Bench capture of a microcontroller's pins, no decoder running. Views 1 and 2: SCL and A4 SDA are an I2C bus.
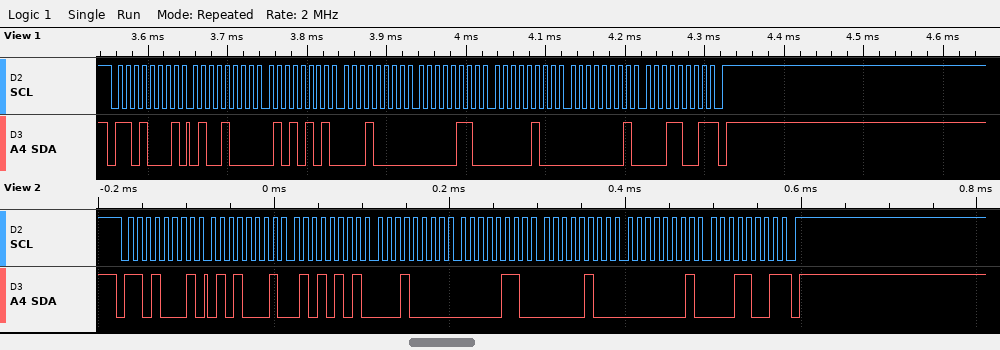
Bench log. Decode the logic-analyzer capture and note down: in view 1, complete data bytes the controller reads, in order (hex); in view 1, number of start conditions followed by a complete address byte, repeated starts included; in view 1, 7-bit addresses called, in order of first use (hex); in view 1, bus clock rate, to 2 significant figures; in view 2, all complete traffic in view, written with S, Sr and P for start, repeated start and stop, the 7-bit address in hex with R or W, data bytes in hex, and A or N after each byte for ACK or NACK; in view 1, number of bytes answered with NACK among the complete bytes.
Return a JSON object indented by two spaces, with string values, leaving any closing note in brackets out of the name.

{
  "in view 1, complete data bytes the controller reads, in order": "48 55 10 06 04 01 19",
  "in view 1, number of start conditions followed by a complete address byte, repeated starts included": "1",
  "in view 1, 7-bit addresses called, in order of first use": "0x68",
  "in view 1, bus clock rate, to 2 significant figures": "100 kHz",
  "in view 2, all complete traffic in view, written with S, Sr and P for start, repeated start and stop, the 7-bit address in hex with R or W, data bytes in hex, and A or N after each byte for ACK or NACK": "S 68R A 51 A 55 A 10 A 06 A 04 A 01 A 19 N P",
  "in view 1, number of bytes answered with NACK among the complete bytes": "1"
}
